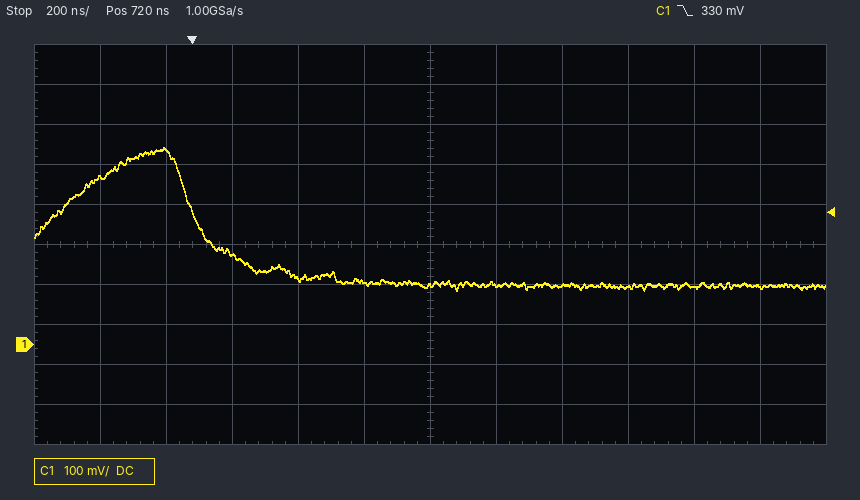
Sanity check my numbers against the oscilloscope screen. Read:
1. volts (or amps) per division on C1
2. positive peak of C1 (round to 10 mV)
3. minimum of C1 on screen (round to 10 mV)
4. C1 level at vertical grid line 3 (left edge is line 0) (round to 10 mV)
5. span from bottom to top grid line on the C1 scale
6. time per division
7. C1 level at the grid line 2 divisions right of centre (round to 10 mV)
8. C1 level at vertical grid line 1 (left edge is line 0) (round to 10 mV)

100 mV
490 mV
140 mV
230 mV
1 V
200 ns
150 mV
420 mV
